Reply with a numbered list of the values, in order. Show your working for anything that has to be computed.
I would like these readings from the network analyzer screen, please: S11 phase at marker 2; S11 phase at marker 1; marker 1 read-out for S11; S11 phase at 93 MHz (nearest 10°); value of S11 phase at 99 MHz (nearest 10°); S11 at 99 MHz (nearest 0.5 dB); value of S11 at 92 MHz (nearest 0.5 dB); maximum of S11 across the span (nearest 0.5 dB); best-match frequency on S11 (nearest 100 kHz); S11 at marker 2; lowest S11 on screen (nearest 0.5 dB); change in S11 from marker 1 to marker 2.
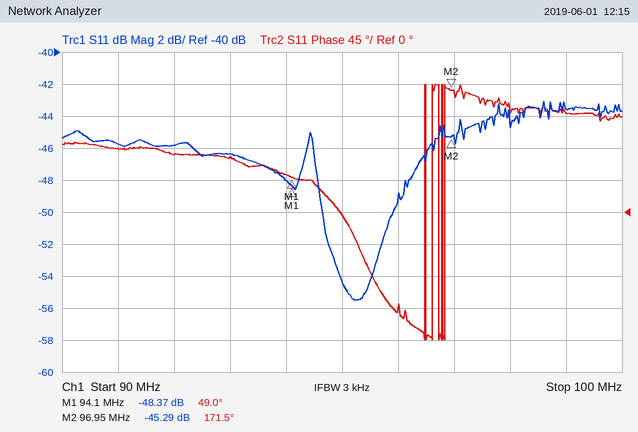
1. 171.5°
2. 49.0°
3. -48.37 dB
4. 80°
5. 140°
6. -43.5 dB
7. -46.0 dB
8. -43.0 dB
9. 95.2 MHz
10. -45.29 dB
11. -55.5 dB
12. -45.29 − (-48.37) = 3.08 dB
